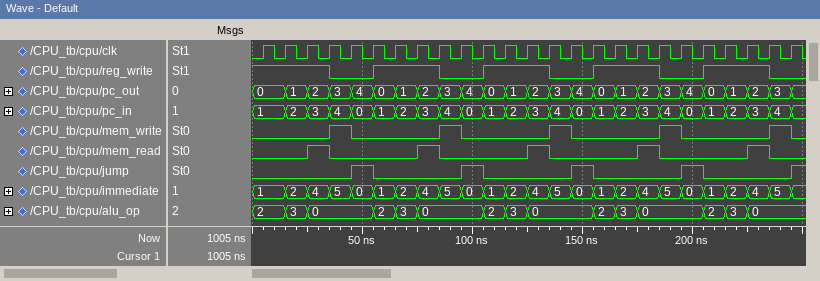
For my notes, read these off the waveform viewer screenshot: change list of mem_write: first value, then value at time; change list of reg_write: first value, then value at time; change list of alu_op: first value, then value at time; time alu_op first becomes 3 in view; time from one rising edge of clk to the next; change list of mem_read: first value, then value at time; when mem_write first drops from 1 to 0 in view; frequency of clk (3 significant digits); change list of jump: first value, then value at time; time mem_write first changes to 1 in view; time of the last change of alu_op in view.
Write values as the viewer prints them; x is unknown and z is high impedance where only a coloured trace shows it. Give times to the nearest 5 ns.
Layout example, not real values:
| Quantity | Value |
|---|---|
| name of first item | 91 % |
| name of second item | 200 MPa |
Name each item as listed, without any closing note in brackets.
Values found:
| Quantity | Value |
|---|---|
| change list of mem_write: first value, then value at time | 0, 1 at 35 ns, 0 at 45 ns, 1 at 85 ns, 0 at 95 ns, 1 at 135 ns, 0 at 145 ns, 1 at 185 ns, 0 at 195 ns, 1 at 235 ns, 0 at 245 ns |
| change list of reg_write: first value, then value at time | 1, 0 at 35 ns, 1 at 55 ns, 0 at 85 ns, 1 at 105 ns, 0 at 135 ns, 1 at 155 ns, 0 at 185 ns, 1 at 205 ns, 0 at 235 ns |
| change list of alu_op: first value, then value at time | 2, 3 at 15 ns, 0 at 25 ns, 2 at 55 ns, 3 at 65 ns, 0 at 75 ns, 2 at 105 ns, 3 at 115 ns, 0 at 125 ns, 2 at 155 ns, 3 at 165 ns, 0 at 175 ns, 2 at 205 ns, 3 at 215 ns, 0 at 225 ns |
| time alu_op first becomes 3 in view | 15 ns |
| time from one rising edge of clk to the next | 10 ns |
| change list of mem_read: first value, then value at time | 0, 1 at 25 ns, 0 at 35 ns, 1 at 75 ns, 0 at 85 ns, 1 at 125 ns, 0 at 135 ns, 1 at 175 ns, 0 at 185 ns, 1 at 225 ns, 0 at 235 ns |
| when mem_write first drops from 1 to 0 in view | 45 ns |
| frequency of clk | 100 MHz |
| change list of jump: first value, then value at time | 0, 1 at 45 ns, 0 at 55 ns, 1 at 95 ns, 0 at 105 ns, 1 at 145 ns, 0 at 155 ns, 1 at 195 ns, 0 at 205 ns, 1 at 245 ns |
| time mem_write first changes to 1 in view | 35 ns |
| time of the last change of alu_op in view | 225 ns |
